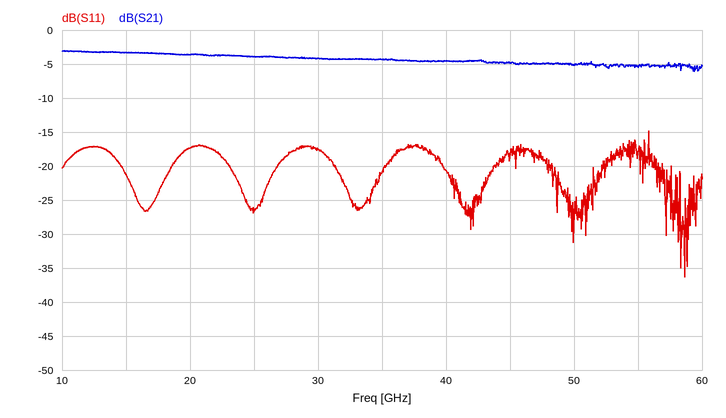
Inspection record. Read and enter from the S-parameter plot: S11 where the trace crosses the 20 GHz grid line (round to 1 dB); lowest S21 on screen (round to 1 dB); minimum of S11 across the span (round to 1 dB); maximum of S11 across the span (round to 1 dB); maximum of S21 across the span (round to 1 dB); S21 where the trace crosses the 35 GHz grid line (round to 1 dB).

-17 dB
-6 dB
-36 dB
-15 dB
-3 dB
-4 dB
